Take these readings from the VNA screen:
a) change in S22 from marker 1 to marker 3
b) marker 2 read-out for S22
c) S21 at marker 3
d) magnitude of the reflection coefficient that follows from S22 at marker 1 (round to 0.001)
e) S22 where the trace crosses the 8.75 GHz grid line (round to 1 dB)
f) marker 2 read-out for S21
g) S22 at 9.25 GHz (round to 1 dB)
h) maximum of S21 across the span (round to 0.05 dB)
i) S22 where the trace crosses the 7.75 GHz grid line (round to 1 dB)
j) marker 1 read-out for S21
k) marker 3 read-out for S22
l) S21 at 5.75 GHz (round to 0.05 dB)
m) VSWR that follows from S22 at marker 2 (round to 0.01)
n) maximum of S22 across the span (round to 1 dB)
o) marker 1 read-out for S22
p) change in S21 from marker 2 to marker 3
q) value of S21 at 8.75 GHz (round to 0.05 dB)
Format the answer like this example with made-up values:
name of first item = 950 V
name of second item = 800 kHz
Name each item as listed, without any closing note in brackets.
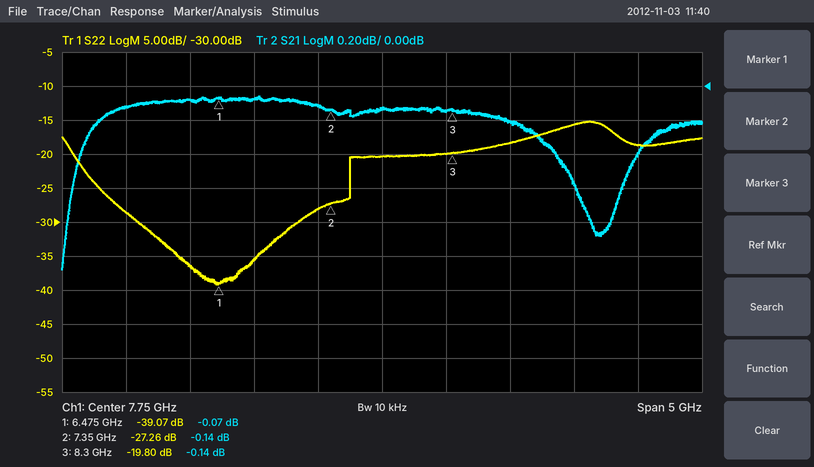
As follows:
change in S22 from marker 1 to marker 3 = 19.27 dB
marker 2 read-out for S22 = -27.26 dB
S21 at marker 3 = -0.14 dB
magnitude of the reflection coefficient that follows from S22 at marker 1 = 0.011
S22 where the trace crosses the 8.75 GHz grid line = -18 dB
marker 2 read-out for S21 = -0.14 dB
S22 at 9.25 GHz = -16 dB
maximum of S21 across the span = -0.05 dB
S22 where the trace crosses the 7.75 GHz grid line = -20 dB
marker 1 read-out for S21 = -0.07 dB
marker 3 read-out for S22 = -19.80 dB
S21 at 5.75 GHz = -0.10 dB
VSWR that follows from S22 at marker 2 = 1.09
maximum of S22 across the span = -15 dB
marker 1 read-out for S22 = -39.07 dB
change in S21 from marker 2 to marker 3 = 0.00 dB
value of S21 at 8.75 GHz = -0.20 dB
